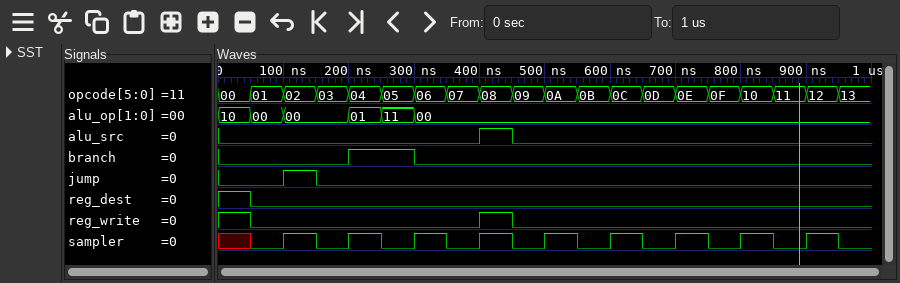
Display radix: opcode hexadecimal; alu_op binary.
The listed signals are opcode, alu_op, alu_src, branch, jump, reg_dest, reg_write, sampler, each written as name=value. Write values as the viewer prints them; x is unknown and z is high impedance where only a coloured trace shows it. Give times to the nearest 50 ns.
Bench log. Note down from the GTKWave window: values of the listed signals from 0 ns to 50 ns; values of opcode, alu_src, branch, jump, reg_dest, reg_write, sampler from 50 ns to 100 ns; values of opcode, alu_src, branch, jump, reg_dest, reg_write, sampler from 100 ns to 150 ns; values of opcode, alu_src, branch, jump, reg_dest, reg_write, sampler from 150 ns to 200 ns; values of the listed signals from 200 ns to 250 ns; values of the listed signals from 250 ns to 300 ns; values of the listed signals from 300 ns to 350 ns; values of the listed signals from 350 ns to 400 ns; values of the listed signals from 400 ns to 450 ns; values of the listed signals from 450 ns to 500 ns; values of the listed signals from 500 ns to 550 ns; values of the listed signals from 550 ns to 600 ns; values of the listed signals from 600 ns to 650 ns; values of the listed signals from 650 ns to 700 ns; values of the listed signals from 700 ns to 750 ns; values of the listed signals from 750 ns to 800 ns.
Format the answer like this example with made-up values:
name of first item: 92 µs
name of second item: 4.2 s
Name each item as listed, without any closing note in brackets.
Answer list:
values of the listed signals from 0 ns to 50 ns: opcode=00, alu_op=10, alu_src=0, branch=0, jump=0, reg_dest=1, reg_write=1, sampler=x
values of opcode, alu_src, branch, jump, reg_dest, reg_write, sampler from 50 ns to 100 ns: opcode=01, alu_src=0, branch=0, jump=0, reg_dest=0, reg_write=0, sampler=0
values of opcode, alu_src, branch, jump, reg_dest, reg_write, sampler from 100 ns to 150 ns: opcode=02, alu_src=0, branch=0, jump=1, reg_dest=0, reg_write=0, sampler=1
values of opcode, alu_src, branch, jump, reg_dest, reg_write, sampler from 150 ns to 200 ns: opcode=03, alu_src=0, branch=0, jump=0, reg_dest=0, reg_write=0, sampler=0
values of the listed signals from 200 ns to 250 ns: opcode=04, alu_op=01, alu_src=0, branch=1, jump=0, reg_dest=0, reg_write=0, sampler=1
values of the listed signals from 250 ns to 300 ns: opcode=05, alu_op=11, alu_src=0, branch=1, jump=0, reg_dest=0, reg_write=0, sampler=0
values of the listed signals from 300 ns to 350 ns: opcode=06, alu_op=00, alu_src=0, branch=0, jump=0, reg_dest=0, reg_write=0, sampler=1
values of the listed signals from 350 ns to 400 ns: opcode=07, alu_op=00, alu_src=0, branch=0, jump=0, reg_dest=0, reg_write=0, sampler=0
values of the listed signals from 400 ns to 450 ns: opcode=08, alu_op=00, alu_src=1, branch=0, jump=0, reg_dest=0, reg_write=1, sampler=1
values of the listed signals from 450 ns to 500 ns: opcode=09, alu_op=00, alu_src=0, branch=0, jump=0, reg_dest=0, reg_write=0, sampler=0
values of the listed signals from 500 ns to 550 ns: opcode=0A, alu_op=00, alu_src=0, branch=0, jump=0, reg_dest=0, reg_write=0, sampler=1
values of the listed signals from 550 ns to 600 ns: opcode=0B, alu_op=00, alu_src=0, branch=0, jump=0, reg_dest=0, reg_write=0, sampler=0
values of the listed signals from 600 ns to 650 ns: opcode=0C, alu_op=00, alu_src=0, branch=0, jump=0, reg_dest=0, reg_write=0, sampler=1
values of the listed signals from 650 ns to 700 ns: opcode=0D, alu_op=00, alu_src=0, branch=0, jump=0, reg_dest=0, reg_write=0, sampler=0
values of the listed signals from 700 ns to 750 ns: opcode=0E, alu_op=00, alu_src=0, branch=0, jump=0, reg_dest=0, reg_write=0, sampler=1
values of the listed signals from 750 ns to 800 ns: opcode=0F, alu_op=00, alu_src=0, branch=0, jump=0, reg_dest=0, reg_write=0, sampler=0
